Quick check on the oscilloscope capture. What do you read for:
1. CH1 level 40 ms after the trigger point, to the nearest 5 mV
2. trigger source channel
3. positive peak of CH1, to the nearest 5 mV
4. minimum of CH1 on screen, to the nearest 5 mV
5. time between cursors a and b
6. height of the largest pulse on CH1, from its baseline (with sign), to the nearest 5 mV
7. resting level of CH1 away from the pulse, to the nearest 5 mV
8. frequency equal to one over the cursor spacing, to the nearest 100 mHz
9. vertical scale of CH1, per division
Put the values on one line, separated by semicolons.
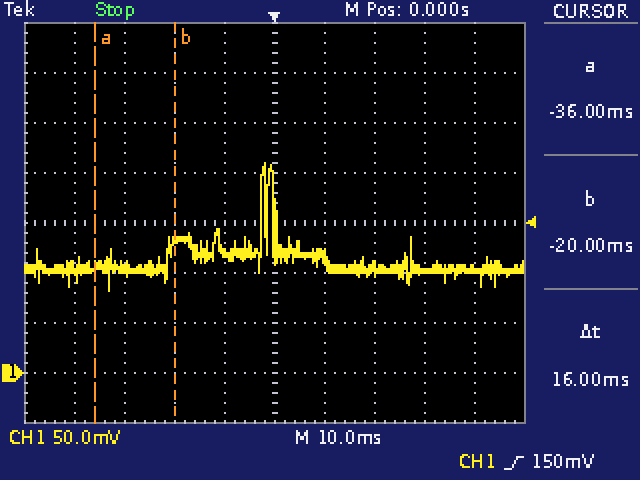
105 mV; CH1; 210 mV; 80 mV; 16 ms; +105 mV; 105 mV; 62.5 Hz; 50 mV
